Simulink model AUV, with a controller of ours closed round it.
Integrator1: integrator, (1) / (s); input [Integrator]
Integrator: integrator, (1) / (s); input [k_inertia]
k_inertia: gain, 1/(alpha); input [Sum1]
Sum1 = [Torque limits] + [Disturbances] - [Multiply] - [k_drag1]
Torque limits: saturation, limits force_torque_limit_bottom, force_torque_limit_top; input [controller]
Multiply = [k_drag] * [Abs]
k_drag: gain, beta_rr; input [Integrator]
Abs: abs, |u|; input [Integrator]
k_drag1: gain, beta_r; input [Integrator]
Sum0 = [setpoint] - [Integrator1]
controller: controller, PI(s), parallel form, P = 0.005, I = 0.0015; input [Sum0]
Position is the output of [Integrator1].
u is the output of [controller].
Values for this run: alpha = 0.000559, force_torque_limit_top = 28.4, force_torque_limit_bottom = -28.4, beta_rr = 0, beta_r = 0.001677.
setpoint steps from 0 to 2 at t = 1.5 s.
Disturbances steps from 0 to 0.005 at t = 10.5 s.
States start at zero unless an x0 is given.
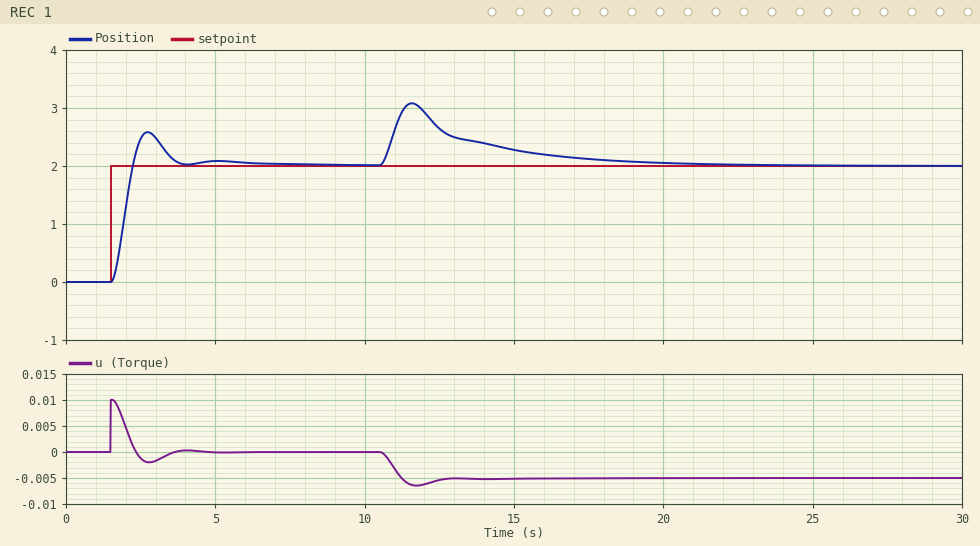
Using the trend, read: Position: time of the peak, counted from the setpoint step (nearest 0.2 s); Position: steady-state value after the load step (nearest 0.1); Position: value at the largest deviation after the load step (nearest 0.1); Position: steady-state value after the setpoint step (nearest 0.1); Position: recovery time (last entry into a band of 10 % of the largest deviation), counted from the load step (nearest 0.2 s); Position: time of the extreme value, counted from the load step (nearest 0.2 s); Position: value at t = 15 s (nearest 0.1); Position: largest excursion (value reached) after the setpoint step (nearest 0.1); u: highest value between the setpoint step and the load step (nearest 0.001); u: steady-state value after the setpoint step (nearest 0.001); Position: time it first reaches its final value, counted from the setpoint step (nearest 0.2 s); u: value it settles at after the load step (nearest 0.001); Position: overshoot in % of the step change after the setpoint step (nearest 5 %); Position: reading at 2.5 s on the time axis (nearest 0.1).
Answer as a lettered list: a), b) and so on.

a) 1.2 s
b) 2.0
c) 3.1
d) 2.0
e) 7.4 s
f) 1.0 s
g) 2.3
h) 2.6
i) 0.010
j) 0.000
k) 0.8 s
l) -0.005
m) 30 %
n) 2.5
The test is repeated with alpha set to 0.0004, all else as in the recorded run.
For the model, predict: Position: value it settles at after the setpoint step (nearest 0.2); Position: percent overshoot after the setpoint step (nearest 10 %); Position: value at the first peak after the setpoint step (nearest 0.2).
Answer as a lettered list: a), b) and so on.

a) 2.0
b) 20 %
c) 2.4
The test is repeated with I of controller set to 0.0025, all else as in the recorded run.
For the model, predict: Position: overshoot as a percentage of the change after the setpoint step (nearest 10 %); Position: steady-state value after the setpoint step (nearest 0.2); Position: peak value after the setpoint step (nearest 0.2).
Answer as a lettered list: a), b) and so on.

a) 40 %
b) 2.0
c) 2.8
